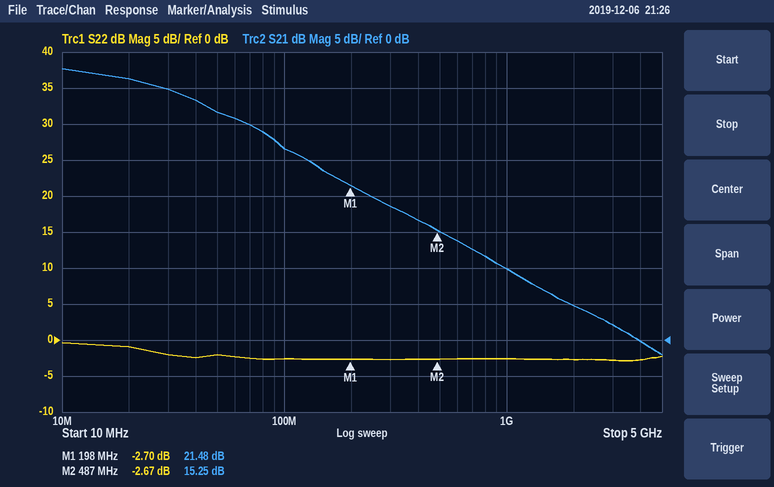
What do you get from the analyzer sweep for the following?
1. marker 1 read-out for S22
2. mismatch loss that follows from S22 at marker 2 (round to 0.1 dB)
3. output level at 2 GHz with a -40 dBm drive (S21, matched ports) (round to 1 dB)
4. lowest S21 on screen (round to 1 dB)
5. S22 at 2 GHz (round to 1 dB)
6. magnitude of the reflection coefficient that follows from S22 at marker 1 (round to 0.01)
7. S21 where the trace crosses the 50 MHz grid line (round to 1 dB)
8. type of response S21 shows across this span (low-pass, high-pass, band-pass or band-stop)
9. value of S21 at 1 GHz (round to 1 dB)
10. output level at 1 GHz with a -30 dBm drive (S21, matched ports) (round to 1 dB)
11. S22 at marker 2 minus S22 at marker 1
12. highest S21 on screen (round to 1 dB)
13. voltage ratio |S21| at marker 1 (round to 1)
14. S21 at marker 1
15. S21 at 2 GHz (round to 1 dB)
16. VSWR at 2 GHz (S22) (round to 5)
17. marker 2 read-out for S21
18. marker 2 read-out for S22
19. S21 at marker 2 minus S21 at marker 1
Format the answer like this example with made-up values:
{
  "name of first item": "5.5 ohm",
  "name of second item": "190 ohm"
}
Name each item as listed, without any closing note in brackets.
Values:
{
  "marker 1 read-out for S22": "-2.70 dB",
  "mismatch loss that follows from S22 at marker 2": "3.4 dB",
  "output level at 2 GHz with a -40 dBm drive (S21, matched ports)": "-35 dBm",
  "lowest S21 on screen": "-2 dB",
  "S22 at 2 GHz": "-3 dB",
  "magnitude of the reflection coefficient that follows from S22 at marker 1": "0.73",
  "S21 where the trace crosses the 50 MHz grid line": "32 dB",
  "type of response S21 shows across this span": "low-pass",
  "value of S21 at 1 GHz": "10 dB",
  "output level at 1 GHz with a -30 dBm drive (S21, matched ports)": "-20 dBm",
  "S22 at marker 2 minus S22 at marker 1": "0.03 dB",
  "highest S21 on screen": "38 dB",
  "voltage ratio |S21| at marker 1": "12",
  "S21 at marker 1": "21.48 dB",
  "S21 at 2 GHz": "5 dB",
  "VSWR at 2 GHz (S22)": "5",
  "marker 2 read-out for S21": "15.25 dB",
  "marker 2 read-out for S22": "-2.67 dB",
  "S21 at marker 2 minus S21 at marker 1": "-6.23 dB"
}
